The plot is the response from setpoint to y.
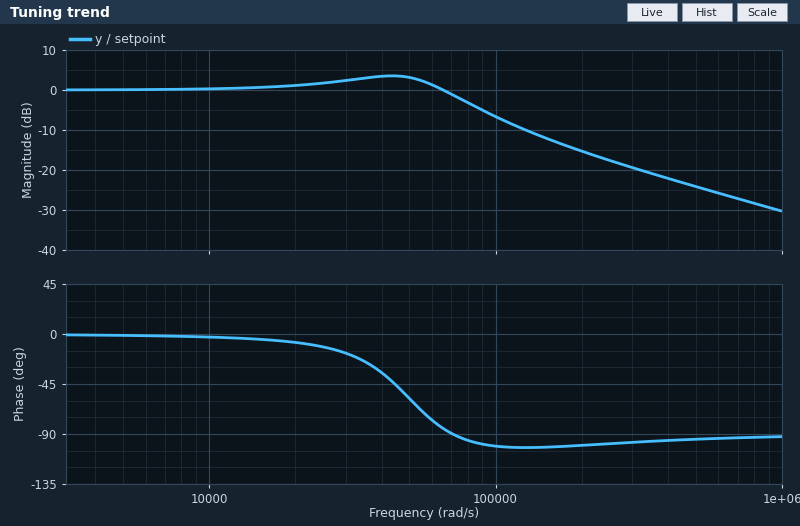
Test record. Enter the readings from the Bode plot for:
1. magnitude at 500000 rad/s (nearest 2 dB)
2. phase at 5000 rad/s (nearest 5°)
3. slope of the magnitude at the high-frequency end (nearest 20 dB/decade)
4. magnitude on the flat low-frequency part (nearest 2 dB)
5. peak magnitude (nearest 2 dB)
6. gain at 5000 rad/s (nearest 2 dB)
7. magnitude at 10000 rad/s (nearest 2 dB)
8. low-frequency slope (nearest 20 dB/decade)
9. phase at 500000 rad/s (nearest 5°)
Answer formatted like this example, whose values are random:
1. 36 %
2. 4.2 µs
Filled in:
1. -24 dB
2. 0°
3. -20 dB/decade
4. 0 dB
5. 4 dB
6. 0 dB
7. 0 dB
8. 0 dB/decade
9. -95°
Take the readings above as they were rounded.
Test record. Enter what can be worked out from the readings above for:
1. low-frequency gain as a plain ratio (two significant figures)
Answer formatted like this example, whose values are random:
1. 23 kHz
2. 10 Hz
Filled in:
1. 1.0
